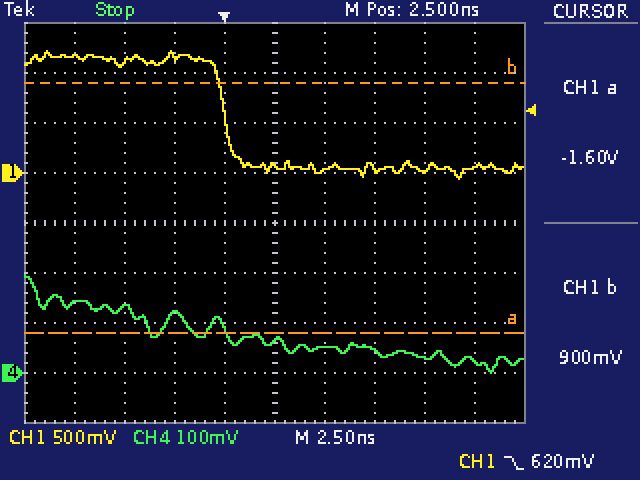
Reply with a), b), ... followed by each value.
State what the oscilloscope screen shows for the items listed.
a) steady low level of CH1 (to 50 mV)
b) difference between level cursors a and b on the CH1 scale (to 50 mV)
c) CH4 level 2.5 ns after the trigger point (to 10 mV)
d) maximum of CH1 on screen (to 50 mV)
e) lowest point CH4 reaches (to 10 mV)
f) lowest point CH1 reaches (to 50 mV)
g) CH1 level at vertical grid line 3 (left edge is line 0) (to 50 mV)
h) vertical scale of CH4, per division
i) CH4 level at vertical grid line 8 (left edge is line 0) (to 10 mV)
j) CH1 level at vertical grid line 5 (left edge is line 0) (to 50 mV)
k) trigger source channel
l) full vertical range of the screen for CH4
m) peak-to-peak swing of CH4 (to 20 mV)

a) 50 mV
b) 2.50 V
c) 60 mV
d) 1.20 V
e) 0 mV
f) -50 mV
g) 1.15 V
h) 100 mV
i) 30 mV
j) 50 mV
k) CH1
l) 800 mV
m) 200 mV
